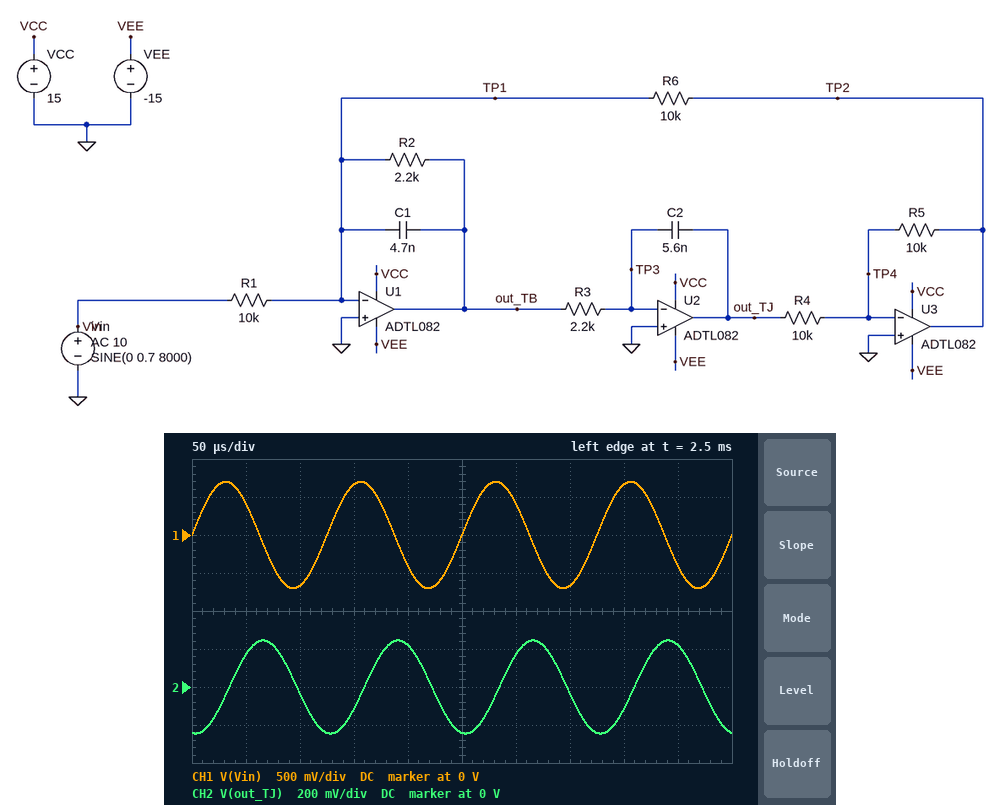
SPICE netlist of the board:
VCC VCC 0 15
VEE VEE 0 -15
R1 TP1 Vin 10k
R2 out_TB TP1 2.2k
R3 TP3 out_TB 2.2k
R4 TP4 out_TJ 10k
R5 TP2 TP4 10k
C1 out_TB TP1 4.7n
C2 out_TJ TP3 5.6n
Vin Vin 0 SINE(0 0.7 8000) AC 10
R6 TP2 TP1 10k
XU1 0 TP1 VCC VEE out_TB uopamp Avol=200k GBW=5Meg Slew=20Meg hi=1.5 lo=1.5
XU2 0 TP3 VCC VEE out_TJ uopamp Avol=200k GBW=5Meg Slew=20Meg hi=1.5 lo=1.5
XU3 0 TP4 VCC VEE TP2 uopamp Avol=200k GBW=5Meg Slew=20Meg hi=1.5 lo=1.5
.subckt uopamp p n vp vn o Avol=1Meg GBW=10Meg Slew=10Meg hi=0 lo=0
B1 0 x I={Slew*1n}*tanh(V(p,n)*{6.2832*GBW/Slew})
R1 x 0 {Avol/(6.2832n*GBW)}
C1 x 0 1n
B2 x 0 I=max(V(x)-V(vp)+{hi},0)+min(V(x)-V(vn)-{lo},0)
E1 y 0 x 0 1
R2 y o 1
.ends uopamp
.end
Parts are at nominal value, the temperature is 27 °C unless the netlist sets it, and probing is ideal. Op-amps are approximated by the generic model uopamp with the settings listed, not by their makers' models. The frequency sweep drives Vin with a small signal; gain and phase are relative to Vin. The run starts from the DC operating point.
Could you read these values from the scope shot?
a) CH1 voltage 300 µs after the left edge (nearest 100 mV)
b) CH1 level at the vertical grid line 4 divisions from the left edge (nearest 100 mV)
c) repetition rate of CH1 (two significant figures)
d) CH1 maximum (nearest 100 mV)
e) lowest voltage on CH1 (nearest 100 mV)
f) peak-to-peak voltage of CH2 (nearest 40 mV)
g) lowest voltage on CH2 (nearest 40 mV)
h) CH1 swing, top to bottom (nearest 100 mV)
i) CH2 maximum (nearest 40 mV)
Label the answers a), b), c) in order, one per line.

a) 400 mV
b) -400 mV
c) 8.0 kHz
d) 700 mV
e) -700 mV
f) 480 mV
g) -240 mV
h) 1.4 V
i) 240 mV
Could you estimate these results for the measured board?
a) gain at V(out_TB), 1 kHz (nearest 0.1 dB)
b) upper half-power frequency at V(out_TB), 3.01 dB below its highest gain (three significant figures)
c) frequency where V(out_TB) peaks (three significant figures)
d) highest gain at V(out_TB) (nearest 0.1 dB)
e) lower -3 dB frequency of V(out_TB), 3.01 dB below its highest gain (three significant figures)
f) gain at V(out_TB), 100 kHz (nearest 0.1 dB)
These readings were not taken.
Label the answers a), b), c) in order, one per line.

a) -22.5 dB
b) 17.8 kHz
c) 6.60 kHz
d) -13.1 dB
e) 2.45 kHz
f) -29.5 dB
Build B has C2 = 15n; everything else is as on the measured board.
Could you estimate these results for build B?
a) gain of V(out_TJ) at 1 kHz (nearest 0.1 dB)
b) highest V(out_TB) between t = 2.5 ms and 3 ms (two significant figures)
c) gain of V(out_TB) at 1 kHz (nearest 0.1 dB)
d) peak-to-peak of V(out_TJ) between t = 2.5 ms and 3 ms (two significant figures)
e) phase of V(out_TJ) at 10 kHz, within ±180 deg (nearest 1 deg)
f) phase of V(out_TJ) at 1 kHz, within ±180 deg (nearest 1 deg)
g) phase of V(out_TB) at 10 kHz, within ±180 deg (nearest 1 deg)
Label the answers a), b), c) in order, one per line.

a) -2.5 dB
b) 140 mV
c) -16.1 dB
d) 170 mV
e) -119 deg
f) -45 deg
g) 151 deg
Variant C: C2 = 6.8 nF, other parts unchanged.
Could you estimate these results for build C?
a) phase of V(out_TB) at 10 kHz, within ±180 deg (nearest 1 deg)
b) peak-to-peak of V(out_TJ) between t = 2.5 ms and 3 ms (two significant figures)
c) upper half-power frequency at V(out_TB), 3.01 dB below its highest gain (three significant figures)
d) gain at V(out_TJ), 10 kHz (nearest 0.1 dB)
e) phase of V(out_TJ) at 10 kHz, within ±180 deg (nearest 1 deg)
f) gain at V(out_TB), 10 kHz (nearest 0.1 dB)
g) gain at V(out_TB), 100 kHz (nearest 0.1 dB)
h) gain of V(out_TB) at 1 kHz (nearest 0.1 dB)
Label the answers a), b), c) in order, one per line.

a) 157 deg
b) 400 mV
c) 17.4 kHz
d) -13.3 dB
e) -113 deg
f) -13.8 dB
g) -29.5 dB
h) -21.0 dB
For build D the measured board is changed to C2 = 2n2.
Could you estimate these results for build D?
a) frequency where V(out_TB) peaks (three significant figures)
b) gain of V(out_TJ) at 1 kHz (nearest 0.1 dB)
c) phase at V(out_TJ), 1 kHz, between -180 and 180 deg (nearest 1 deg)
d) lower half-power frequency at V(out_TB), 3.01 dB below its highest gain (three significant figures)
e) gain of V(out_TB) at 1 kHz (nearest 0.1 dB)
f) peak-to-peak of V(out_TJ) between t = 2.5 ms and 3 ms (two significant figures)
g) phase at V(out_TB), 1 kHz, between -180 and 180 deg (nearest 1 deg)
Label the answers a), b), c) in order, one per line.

a) 10.5 kHz
b) 0 dB
c) -8 deg
d) 5.35 kHz
e) -30.3 dB
f) 1.2 V
g) -98 deg
